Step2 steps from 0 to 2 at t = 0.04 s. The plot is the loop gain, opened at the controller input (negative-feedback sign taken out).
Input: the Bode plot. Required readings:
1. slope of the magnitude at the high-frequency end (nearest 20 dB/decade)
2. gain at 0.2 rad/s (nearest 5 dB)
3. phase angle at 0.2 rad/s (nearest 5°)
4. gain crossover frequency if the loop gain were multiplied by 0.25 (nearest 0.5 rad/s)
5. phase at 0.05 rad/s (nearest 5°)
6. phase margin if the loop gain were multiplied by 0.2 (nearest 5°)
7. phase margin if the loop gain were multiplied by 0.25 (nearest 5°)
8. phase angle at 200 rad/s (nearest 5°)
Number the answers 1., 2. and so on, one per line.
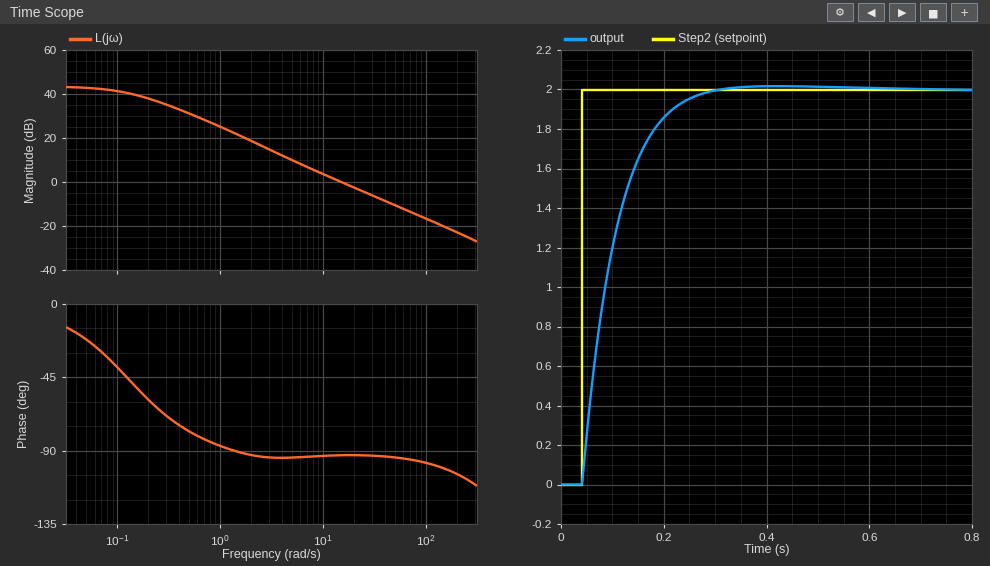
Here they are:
1. -20 dB/decade
2. 40 dB
3. -60°
4. 4.0 rad/s
5. -20°
6. 85°
7. 85°
8. -105°
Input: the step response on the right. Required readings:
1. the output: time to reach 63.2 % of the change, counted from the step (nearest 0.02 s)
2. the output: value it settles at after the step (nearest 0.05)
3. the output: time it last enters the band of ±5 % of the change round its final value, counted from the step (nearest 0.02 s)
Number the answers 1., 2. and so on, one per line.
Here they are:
1. 0.06 s
2. 2.00
3. 0.18 s
